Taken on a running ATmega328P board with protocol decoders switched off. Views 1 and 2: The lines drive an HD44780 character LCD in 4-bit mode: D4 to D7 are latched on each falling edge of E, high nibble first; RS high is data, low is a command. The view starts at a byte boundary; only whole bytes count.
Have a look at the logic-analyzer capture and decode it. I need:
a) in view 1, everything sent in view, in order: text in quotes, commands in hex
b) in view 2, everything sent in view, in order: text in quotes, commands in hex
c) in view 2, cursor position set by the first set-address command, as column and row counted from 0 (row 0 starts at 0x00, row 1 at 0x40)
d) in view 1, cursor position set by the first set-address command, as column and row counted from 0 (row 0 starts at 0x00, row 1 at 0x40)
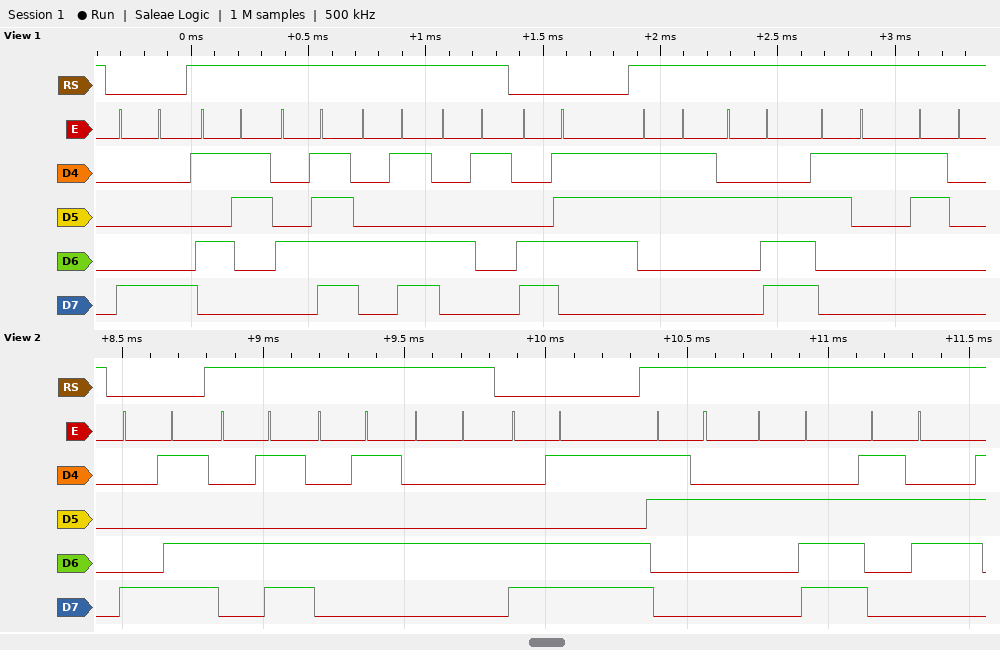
0x88 "SOMA" 0xC7 "3.10"
0x8D "MED" 0xCD "2.6"
column 13, row 0
column 8, row 0
